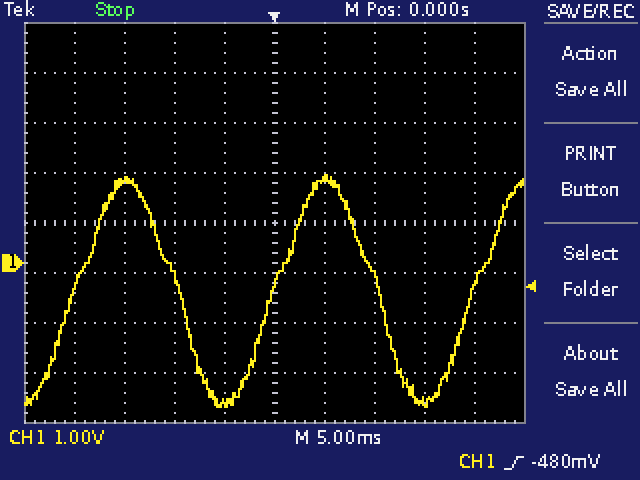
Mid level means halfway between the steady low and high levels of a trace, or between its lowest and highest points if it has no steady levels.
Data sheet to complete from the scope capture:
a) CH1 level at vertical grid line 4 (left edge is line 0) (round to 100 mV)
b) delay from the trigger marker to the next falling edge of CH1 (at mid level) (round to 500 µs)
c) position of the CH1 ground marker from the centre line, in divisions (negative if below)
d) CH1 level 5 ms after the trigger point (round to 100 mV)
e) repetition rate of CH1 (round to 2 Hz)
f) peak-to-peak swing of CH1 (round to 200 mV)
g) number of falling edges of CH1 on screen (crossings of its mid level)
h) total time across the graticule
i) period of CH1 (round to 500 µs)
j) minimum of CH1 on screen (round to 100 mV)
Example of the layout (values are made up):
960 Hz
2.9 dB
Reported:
-2.8 V
10.5 ms
-0.8 div
1.7 V
50 Hz
4.6 V
2
50 ms
20.0 ms
-2.9 V
